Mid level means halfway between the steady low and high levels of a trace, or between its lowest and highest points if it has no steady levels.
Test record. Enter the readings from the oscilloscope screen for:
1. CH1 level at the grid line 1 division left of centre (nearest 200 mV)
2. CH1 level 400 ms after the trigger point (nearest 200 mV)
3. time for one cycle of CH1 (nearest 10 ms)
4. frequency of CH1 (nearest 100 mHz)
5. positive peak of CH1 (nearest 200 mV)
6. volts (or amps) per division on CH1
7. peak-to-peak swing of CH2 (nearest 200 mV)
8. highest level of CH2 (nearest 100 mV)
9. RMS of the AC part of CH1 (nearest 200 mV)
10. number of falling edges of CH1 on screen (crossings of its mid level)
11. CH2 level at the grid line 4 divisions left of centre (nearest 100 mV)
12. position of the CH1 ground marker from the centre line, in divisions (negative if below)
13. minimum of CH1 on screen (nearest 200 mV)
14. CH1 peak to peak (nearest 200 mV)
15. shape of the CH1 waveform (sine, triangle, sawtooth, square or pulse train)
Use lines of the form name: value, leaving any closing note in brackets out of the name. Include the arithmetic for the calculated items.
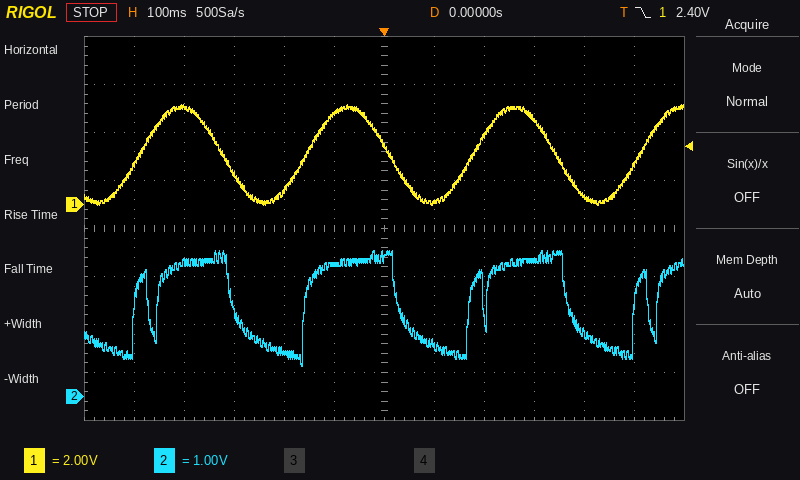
CH1 level at the grid line 1 division left of centre: 3.8 V
CH1 level 400 ms after the trigger point: 400 mV
time for one cycle of CH1: 330 ms
frequency of CH1: 1 / 330 ms ≈ 3.0 Hz
positive peak of CH1: 4.2 V
volts (or amps) per division on CH1: 2 V
peak-to-peak swing of CH2: 2.4 V
highest level of CH2: 3.0 V
RMS of the AC part of CH1: 4.2 V / (2√2) ≈ 1.48 V, so 1.4 V to the nearest 200 mV
number of falling edges of CH1 on screen: 3
CH2 level at the grid line 4 divisions left of centre: 2.8 V
position of the CH1 ground marker from the centre line, in divisions: +0.5 div
minimum of CH1 on screen: 0.0 V
CH1 peak to peak: 4.2 V − (0.0 V) = 4.2 V
shape of the CH1 waveform: sine
